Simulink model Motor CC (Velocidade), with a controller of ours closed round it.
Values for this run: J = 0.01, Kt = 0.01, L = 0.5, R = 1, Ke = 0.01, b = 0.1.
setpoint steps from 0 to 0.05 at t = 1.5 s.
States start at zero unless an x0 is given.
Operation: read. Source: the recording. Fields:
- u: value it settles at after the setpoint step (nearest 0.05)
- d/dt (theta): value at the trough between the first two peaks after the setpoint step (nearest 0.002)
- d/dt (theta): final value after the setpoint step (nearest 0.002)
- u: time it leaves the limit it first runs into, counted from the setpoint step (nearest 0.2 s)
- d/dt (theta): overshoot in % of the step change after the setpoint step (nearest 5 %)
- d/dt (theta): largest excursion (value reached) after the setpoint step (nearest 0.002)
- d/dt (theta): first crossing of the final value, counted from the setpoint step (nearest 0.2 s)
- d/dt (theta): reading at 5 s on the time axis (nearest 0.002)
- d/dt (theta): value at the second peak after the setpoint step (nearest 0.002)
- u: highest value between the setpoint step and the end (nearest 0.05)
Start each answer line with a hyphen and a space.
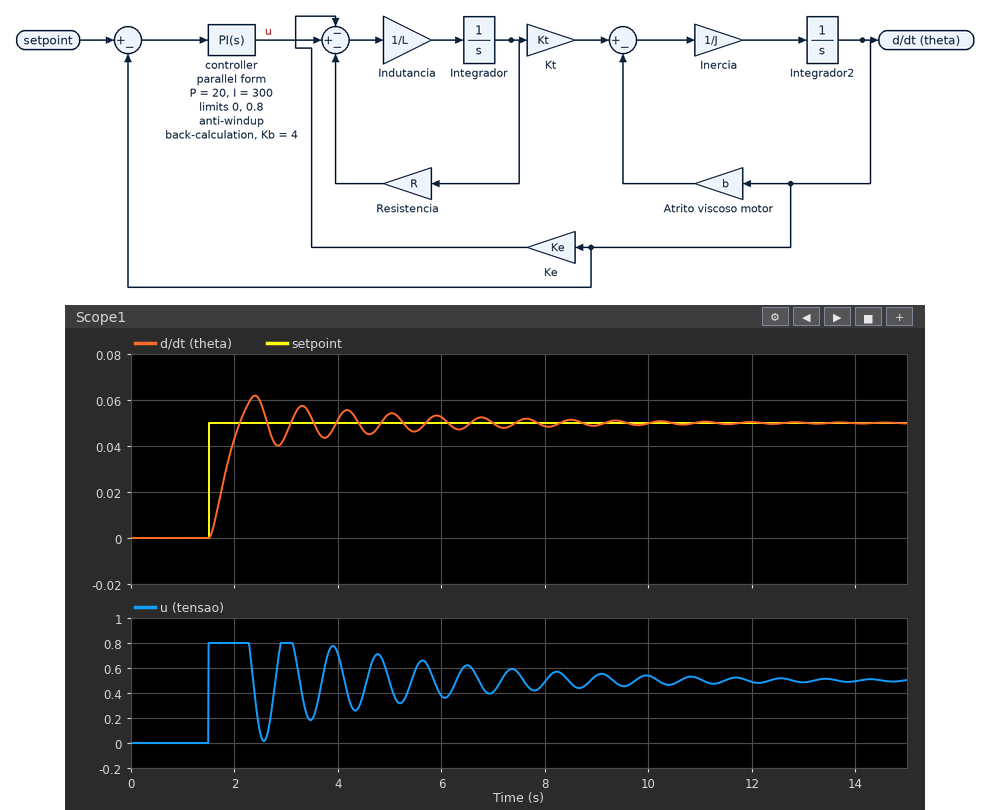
- 0.50
- 0.040
- 0.050
- 0.8 s
- 25 %
- 0.062
- 0.6 s
- 0.054
- 0.058
- 0.80
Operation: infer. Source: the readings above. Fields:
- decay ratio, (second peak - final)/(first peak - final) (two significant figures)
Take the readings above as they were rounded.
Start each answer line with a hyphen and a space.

- 0.67
